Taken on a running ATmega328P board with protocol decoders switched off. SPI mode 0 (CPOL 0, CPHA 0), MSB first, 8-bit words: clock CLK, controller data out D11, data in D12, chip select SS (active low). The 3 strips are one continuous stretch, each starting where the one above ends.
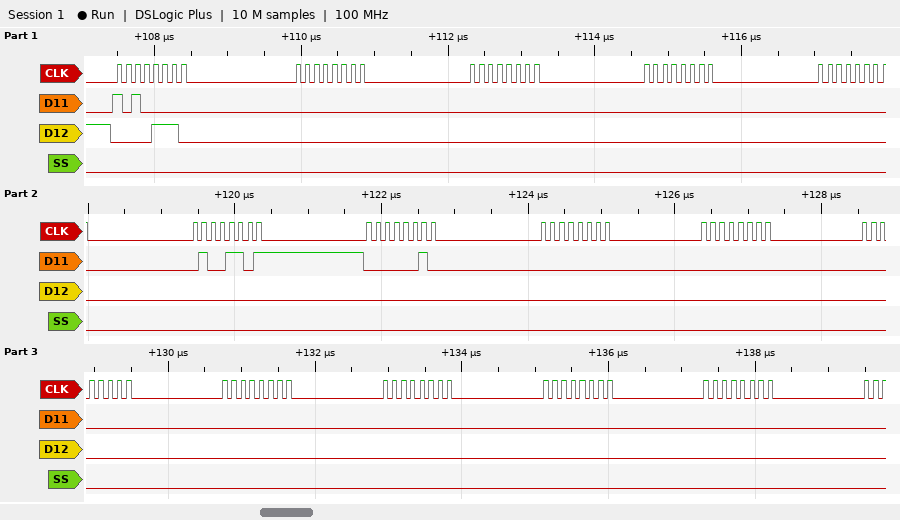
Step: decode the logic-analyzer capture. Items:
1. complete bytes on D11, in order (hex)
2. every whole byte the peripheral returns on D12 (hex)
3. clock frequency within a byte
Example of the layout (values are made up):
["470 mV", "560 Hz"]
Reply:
["A0 00 00 00 00 4D 02 00 00 00 00 00 00 00", "0E 00 00 00 00 00 00 00 00 00 00 00 00 00", "8 MHz"]
